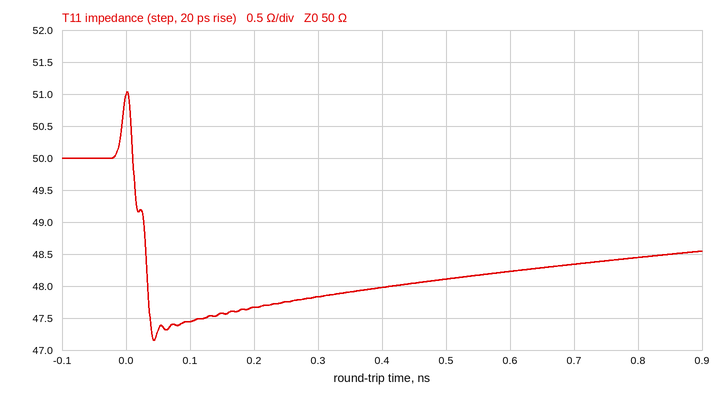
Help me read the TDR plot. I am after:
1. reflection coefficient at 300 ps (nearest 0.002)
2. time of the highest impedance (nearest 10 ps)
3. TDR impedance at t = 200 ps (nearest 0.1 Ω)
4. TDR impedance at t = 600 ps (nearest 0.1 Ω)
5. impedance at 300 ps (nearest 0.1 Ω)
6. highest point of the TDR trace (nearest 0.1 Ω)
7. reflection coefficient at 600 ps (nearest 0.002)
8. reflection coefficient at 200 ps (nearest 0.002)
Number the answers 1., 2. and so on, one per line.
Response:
1. -0.022
2. 0 ps
3. 47.7 Ω
4. 48.2 Ω
5. 47.8 Ω
6. 51.0 Ω
7. -0.018
8. -0.024
